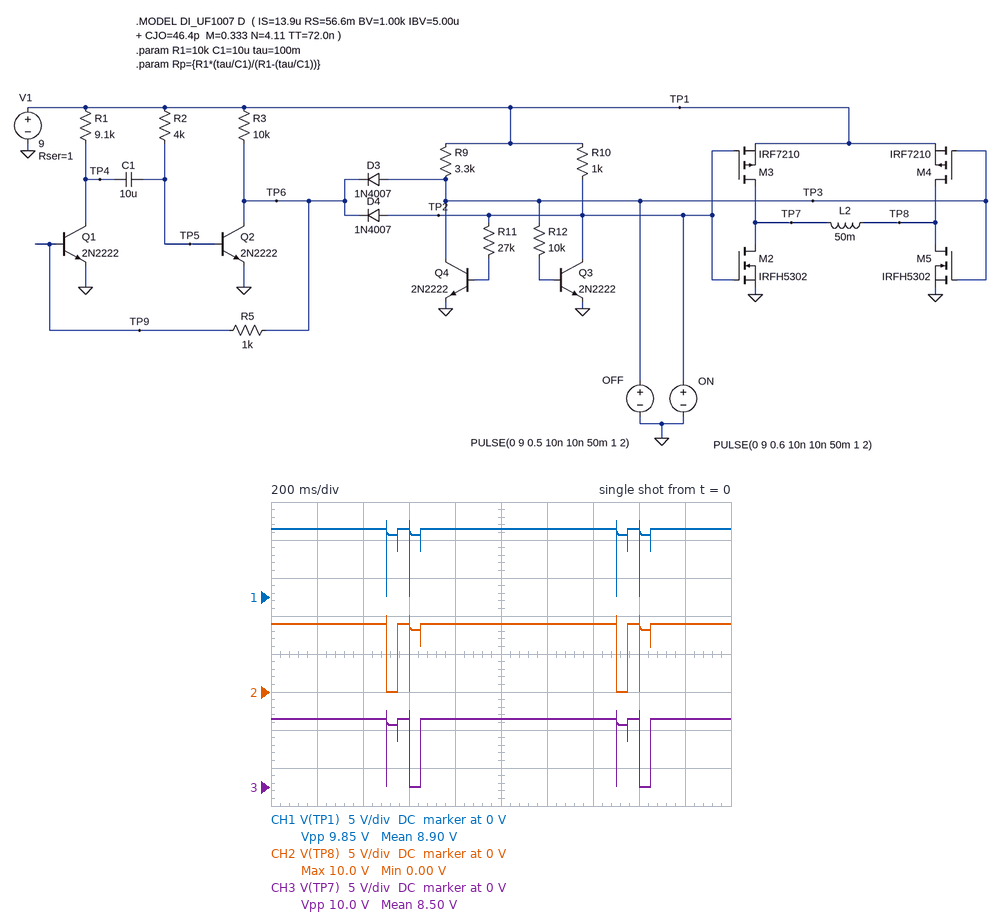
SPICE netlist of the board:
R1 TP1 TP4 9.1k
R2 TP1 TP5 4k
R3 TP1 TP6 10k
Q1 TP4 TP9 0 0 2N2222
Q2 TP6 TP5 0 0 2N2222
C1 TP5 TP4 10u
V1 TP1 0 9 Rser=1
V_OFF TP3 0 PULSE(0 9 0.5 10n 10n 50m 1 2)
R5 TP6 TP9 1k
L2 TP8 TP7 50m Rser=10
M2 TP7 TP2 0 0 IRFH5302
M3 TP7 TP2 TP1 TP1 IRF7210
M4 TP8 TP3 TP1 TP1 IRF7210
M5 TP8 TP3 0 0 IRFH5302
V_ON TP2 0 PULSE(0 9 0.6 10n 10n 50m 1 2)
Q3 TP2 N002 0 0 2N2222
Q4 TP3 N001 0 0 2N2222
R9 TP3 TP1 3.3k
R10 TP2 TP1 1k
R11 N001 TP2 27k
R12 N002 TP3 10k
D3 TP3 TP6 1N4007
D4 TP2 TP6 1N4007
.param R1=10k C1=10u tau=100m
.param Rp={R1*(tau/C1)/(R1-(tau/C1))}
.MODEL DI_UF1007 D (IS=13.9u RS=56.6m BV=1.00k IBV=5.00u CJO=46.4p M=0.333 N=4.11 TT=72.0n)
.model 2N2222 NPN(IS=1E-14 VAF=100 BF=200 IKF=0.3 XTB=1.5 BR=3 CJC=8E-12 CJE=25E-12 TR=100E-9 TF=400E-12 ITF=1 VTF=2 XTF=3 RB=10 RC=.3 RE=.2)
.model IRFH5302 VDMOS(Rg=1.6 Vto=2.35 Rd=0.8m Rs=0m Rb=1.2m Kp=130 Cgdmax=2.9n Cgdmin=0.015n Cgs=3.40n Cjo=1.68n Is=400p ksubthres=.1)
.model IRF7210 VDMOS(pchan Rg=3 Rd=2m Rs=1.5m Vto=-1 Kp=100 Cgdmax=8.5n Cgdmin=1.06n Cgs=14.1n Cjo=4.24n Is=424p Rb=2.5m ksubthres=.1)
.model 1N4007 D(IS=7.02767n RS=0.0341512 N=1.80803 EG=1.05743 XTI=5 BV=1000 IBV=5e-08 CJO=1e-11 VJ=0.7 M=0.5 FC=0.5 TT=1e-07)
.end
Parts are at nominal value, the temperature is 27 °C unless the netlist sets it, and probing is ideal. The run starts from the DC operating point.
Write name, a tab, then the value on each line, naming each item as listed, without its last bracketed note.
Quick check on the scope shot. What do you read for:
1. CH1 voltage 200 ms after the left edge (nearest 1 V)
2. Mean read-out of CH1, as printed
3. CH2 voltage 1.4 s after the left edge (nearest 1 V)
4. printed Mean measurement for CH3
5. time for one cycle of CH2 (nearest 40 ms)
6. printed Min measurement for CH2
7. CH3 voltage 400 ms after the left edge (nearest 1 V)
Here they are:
CH1 voltage 200 ms after the left edge	9 V
Mean read-out of CH1, as printed	8.90 V
CH2 voltage 1.4 s after the left edge	9 V
printed Mean measurement for CH3	8.50 V
time for one cycle of CH2	1.00 s
printed Min measurement for CH2	0.00 V
CH3 voltage 400 ms after the left edge	9 V
